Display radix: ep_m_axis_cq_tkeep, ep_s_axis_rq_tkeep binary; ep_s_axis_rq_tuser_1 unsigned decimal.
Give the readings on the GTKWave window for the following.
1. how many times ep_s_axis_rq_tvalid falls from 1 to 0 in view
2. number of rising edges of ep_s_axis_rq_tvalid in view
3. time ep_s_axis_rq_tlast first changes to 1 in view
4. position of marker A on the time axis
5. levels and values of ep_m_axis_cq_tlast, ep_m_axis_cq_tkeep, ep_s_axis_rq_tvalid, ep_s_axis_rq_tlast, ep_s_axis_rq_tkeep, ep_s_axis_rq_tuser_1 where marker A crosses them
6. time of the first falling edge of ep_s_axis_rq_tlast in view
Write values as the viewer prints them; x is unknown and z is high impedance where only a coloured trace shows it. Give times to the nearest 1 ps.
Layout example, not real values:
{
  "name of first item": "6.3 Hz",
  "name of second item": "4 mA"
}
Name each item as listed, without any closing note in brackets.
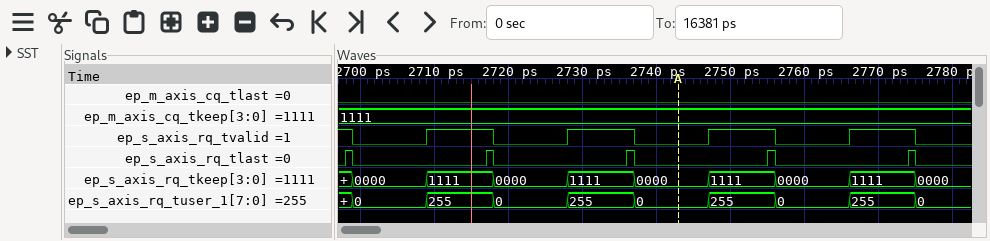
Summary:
{
  "how many times ep_s_axis_rq_tvalid falls from 1 to 0 in view": "5",
  "number of rising edges of ep_s_axis_rq_tvalid in view": "4",
  "time ep_s_axis_rq_tlast first changes to 1 in view": "2698 ps",
  "position of marker A on the time axis": "2743 ps",
  "levels and values of ep_m_axis_cq_tlast, ep_m_axis_cq_tkeep, ep_s_axis_rq_tvalid, ep_s_axis_rq_tlast, ep_s_axis_rq_tkeep, ep_s_axis_rq_tuser_1 where marker A crosses them": "ep_m_axis_cq_tlast=0, ep_m_axis_cq_tkeep=1111, ep_s_axis_rq_tvalid=0, ep_s_axis_rq_tlast=0, ep_s_axis_rq_tkeep=0000, ep_s_axis_rq_tuser_1=0",
  "time of the first falling edge of ep_s_axis_rq_tlast in view": "2699 ps"
}
